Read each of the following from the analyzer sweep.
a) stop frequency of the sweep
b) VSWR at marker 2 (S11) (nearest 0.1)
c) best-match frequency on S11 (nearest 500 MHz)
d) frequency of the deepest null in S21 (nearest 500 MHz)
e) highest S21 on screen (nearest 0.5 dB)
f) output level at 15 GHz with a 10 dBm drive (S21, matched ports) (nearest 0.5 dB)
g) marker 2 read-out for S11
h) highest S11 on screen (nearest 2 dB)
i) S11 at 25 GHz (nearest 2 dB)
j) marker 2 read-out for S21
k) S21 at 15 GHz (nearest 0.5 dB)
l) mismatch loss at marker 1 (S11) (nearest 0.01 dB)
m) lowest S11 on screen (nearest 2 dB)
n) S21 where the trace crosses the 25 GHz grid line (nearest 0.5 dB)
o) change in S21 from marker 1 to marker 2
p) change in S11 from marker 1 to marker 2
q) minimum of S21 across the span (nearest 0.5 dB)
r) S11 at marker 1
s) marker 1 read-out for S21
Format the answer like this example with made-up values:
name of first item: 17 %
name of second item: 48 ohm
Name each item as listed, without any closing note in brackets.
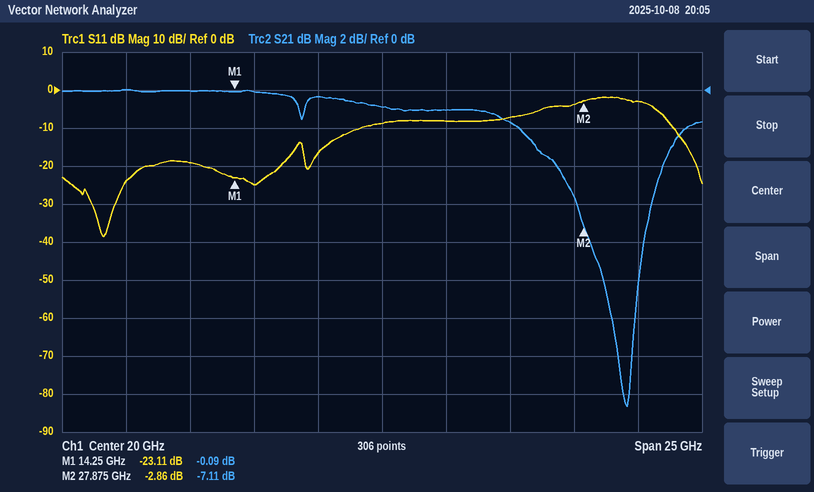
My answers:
stop frequency of the sweep: 32.5 GHz
VSWR at marker 2 (S11): 6.1
best-match frequency on S11: 9.0 GHz
frequency of the deepest null in S21: 29.5 GHz
highest S21 on screen: 0.0 dB
output level at 15 GHz with a 10 dBm drive (S21, matched ports): 10.0 dBm
marker 2 read-out for S11: -2.86 dB
highest S11 on screen: -2 dB
S11 at 25 GHz: -8 dB
marker 2 read-out for S21: -7.11 dB
S21 at 15 GHz: 0.0 dB
mismatch loss at marker 1 (S11): 0.02 dB
lowest S11 on screen: -38 dB
S21 where the trace crosses the 25 GHz grid line: -1.5 dB
change in S21 from marker 1 to marker 2: -7.02 dB
change in S11 from marker 1 to marker 2: 20.25 dB
minimum of S21 across the span: -16.5 dB
S11 at marker 1: -23.11 dB
marker 1 read-out for S21: -0.09 dB
